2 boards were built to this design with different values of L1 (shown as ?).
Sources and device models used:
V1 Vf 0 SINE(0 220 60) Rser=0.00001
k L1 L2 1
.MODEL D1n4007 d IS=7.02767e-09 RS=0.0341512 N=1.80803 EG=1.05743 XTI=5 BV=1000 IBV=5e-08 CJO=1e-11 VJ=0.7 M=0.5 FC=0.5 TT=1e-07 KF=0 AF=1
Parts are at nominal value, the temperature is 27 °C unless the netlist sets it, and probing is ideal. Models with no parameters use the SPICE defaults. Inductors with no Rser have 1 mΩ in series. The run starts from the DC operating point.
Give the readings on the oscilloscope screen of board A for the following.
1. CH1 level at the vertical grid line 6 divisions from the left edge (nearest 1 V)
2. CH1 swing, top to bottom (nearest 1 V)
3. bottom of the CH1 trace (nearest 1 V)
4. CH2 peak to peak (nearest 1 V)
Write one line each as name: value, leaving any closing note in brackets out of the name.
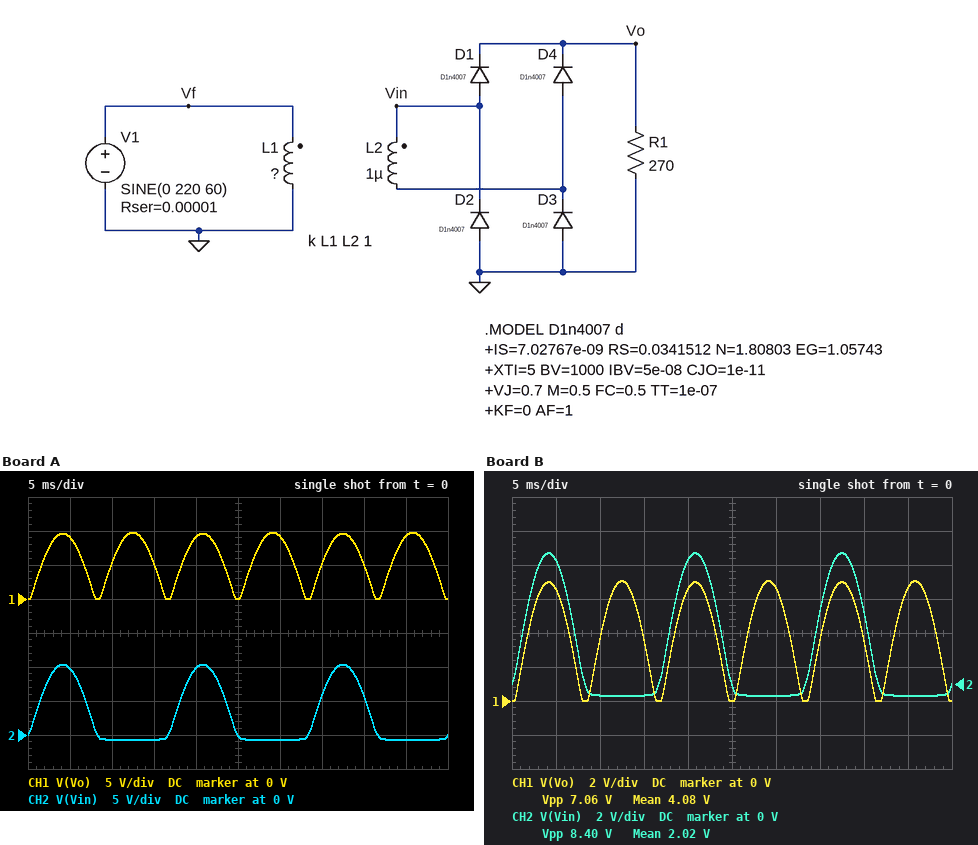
CH1 level at the vertical grid line 6 divisions from the left edge: 9 V
CH1 swing, top to bottom: 10 V
bottom of the CH1 trace: 0 V
CH2 peak to peak: 11 V
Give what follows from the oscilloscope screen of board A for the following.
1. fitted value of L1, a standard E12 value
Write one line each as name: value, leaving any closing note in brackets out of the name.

fitted value of L1, a standard E12 value: 390 µH
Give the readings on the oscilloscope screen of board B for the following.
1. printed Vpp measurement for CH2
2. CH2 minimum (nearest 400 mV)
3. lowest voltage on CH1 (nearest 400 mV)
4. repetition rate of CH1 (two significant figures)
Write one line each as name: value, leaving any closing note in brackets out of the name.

printed Vpp measurement for CH2: 8.40 V
CH2 minimum: -800 mV
lowest voltage on CH1: 0 V
repetition rate of CH1: 120 Hz
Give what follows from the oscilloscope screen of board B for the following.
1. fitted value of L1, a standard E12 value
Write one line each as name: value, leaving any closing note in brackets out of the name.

fitted value of L1, a standard E12 value: 680 µH
